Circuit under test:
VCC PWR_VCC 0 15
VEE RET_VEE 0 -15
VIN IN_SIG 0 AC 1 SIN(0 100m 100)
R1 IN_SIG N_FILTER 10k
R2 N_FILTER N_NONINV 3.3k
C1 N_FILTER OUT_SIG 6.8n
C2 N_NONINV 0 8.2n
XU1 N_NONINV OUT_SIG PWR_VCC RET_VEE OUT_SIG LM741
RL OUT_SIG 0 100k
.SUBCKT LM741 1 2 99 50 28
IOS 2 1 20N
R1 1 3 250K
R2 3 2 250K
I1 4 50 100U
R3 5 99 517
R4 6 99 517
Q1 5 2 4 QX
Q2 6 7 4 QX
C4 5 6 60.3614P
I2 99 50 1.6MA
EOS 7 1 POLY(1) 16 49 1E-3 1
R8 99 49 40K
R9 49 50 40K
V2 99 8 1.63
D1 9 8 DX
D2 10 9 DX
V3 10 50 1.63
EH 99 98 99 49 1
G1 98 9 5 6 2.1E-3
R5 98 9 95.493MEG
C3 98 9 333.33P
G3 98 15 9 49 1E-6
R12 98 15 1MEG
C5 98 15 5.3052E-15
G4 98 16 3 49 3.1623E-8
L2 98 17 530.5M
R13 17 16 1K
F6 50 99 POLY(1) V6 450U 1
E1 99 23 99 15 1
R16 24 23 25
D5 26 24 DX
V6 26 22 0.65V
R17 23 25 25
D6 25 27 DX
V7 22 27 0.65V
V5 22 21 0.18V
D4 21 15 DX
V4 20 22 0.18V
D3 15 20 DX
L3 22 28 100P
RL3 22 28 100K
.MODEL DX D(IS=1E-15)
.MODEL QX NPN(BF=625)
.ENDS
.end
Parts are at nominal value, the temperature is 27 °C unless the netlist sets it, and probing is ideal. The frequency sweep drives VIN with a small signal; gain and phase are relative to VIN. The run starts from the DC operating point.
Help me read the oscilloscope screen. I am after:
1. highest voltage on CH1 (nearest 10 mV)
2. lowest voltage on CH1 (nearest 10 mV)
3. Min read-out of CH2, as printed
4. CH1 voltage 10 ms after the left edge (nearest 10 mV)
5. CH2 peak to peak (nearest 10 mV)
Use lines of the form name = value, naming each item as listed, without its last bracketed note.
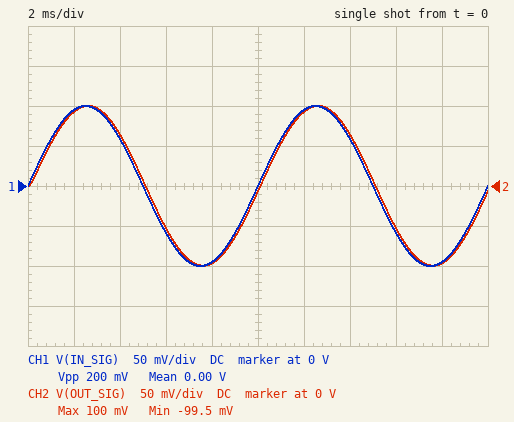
highest voltage on CH1 = 100 mV
lowest voltage on CH1 = -100 mV
Min read-out of CH2, as printed = -99.5 mV
CH1 voltage 10 ms after the left edge = 0 V
CH2 peak to peak = 200 mV
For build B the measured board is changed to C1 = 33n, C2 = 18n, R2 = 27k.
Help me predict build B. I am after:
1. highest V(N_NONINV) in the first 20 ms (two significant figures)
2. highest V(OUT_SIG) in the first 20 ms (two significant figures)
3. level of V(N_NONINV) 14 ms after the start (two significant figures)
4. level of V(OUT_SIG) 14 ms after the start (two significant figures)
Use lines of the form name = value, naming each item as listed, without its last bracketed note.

highest V(N_NONINV) in the first 20 ms = 95 mV
highest V(OUT_SIG) in the first 20 ms = 96 mV
level of V(N_NONINV) 14 ms after the start = 82 mV
level of V(OUT_SIG) 14 ms after the start = 83 mV
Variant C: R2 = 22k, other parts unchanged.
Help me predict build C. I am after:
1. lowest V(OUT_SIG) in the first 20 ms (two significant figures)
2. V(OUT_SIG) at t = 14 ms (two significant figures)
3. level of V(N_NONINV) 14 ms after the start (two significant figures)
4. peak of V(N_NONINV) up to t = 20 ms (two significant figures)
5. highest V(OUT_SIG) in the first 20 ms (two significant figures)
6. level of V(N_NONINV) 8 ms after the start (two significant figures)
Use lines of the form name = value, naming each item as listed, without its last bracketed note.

lowest V(OUT_SIG) in the first 20 ms = -100 mV
V(OUT_SIG) at t = 14 ms = 70 mV
level of V(N_NONINV) 14 ms after the start = 69 mV
peak of V(N_NONINV) up to t = 20 ms = 97 mV
highest V(OUT_SIG) in the first 20 ms = 98 mV
level of V(N_NONINV) 8 ms after the start = -100 mV
